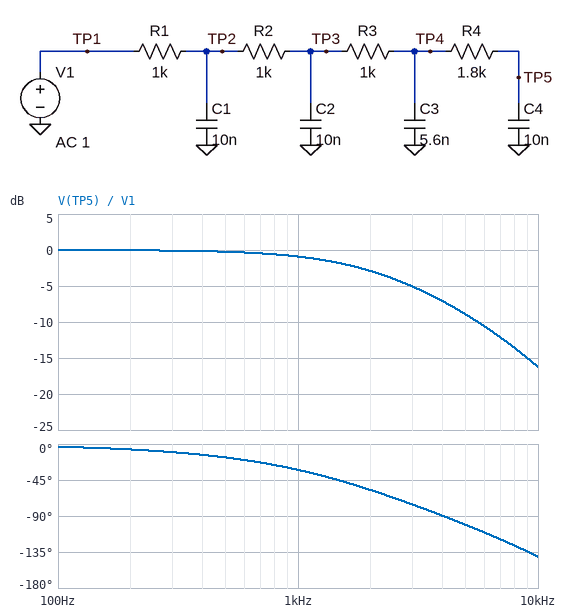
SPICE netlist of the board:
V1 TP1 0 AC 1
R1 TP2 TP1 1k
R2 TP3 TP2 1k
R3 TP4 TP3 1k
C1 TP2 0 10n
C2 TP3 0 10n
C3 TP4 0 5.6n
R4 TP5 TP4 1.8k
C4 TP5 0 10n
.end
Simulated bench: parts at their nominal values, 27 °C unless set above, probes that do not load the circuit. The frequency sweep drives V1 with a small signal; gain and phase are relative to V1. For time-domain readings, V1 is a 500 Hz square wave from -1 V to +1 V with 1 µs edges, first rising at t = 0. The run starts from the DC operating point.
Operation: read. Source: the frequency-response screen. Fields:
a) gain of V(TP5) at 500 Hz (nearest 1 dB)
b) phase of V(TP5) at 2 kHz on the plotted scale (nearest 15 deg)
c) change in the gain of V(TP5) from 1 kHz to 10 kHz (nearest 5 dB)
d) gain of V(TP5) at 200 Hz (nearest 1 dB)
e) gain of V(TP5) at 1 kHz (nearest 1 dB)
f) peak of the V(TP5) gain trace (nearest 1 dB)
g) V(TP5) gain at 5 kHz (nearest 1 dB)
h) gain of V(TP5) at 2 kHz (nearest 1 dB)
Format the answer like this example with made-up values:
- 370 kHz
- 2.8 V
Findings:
- 0 dB
- -60 deg
- -15 dB
- 0 dB
- -1 dB
- 0 dB
- -9 dB
- -3 dB
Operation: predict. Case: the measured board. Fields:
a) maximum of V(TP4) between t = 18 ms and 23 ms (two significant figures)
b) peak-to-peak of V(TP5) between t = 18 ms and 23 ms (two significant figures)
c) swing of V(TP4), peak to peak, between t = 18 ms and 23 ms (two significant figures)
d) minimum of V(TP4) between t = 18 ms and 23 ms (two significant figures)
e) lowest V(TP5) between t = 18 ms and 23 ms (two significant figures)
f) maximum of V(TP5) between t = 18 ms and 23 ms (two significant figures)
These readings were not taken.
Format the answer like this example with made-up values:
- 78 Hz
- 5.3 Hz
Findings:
- 1.0 V
- 2.0 V
- 2.0 V
- -1.0 V
- -1.0 V
- 1.0 V
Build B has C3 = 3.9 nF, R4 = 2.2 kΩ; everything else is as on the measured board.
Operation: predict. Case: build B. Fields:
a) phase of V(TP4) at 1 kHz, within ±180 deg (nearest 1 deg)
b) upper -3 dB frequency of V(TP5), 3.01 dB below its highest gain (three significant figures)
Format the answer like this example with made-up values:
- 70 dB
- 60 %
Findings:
- -24 deg
- 2.08 kHz
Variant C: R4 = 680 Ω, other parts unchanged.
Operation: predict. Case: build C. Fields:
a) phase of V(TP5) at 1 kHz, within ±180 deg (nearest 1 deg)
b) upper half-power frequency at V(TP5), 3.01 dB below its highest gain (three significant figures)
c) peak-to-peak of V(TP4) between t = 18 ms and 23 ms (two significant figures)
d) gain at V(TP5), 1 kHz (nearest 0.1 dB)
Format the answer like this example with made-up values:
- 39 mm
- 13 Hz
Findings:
- -29 deg
- 2.25 kHz
- 2.0 V
- -0.8 dB
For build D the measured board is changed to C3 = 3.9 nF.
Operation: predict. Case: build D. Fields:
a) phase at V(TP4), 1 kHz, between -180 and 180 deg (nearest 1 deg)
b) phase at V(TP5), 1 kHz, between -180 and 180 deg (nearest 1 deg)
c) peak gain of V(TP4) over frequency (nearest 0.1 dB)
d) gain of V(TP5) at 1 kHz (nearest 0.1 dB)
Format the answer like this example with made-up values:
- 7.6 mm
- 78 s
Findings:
- -24 deg
- -31 deg
- 0 dB
- -0.8 dB
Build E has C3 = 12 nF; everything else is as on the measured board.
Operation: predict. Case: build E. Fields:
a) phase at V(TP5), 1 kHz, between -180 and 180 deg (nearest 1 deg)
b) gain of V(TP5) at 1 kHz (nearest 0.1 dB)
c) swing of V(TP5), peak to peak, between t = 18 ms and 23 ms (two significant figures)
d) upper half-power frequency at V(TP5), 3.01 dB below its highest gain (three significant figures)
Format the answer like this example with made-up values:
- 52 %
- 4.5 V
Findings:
- -38 deg
- -1.3 dB
- 2.0 V
- 1.69 kHz
